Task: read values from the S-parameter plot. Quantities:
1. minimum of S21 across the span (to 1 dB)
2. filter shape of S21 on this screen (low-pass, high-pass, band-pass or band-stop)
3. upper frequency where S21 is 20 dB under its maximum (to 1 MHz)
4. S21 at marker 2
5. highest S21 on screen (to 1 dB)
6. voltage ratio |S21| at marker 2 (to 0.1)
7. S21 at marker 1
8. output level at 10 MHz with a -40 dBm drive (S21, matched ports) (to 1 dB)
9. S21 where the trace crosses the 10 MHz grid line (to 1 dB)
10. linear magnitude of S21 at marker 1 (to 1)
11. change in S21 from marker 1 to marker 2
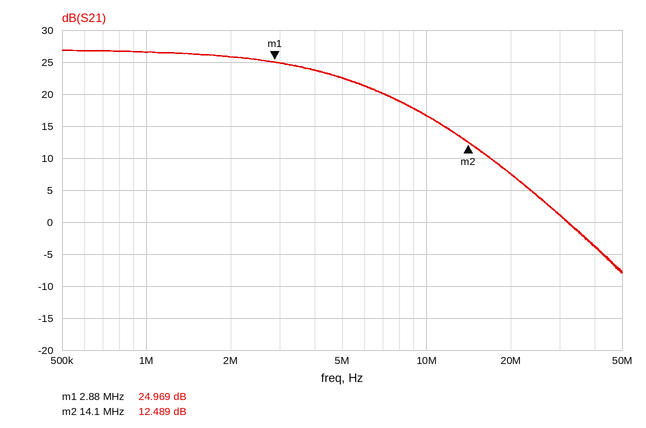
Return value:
-8 dB
low-pass
21 MHz
12.489 dB
27 dB
4.2
24.969 dB
-23 dBm
17 dB
18
-12.480 dB
